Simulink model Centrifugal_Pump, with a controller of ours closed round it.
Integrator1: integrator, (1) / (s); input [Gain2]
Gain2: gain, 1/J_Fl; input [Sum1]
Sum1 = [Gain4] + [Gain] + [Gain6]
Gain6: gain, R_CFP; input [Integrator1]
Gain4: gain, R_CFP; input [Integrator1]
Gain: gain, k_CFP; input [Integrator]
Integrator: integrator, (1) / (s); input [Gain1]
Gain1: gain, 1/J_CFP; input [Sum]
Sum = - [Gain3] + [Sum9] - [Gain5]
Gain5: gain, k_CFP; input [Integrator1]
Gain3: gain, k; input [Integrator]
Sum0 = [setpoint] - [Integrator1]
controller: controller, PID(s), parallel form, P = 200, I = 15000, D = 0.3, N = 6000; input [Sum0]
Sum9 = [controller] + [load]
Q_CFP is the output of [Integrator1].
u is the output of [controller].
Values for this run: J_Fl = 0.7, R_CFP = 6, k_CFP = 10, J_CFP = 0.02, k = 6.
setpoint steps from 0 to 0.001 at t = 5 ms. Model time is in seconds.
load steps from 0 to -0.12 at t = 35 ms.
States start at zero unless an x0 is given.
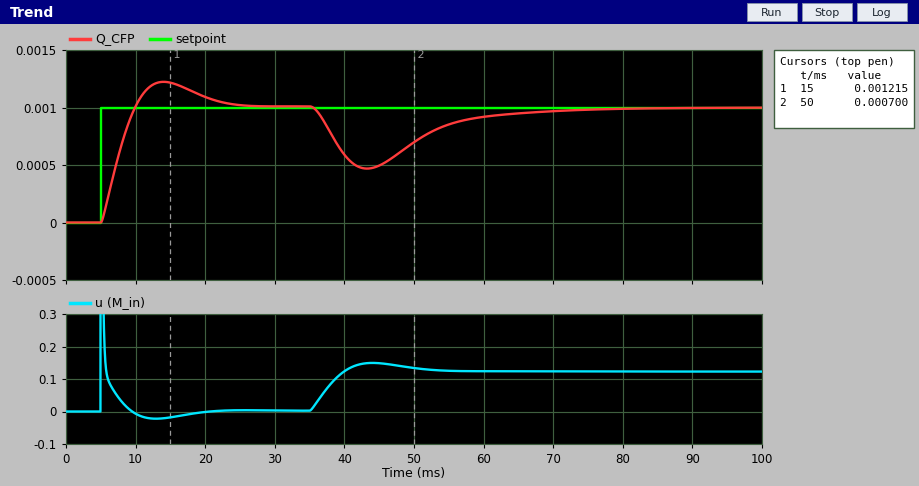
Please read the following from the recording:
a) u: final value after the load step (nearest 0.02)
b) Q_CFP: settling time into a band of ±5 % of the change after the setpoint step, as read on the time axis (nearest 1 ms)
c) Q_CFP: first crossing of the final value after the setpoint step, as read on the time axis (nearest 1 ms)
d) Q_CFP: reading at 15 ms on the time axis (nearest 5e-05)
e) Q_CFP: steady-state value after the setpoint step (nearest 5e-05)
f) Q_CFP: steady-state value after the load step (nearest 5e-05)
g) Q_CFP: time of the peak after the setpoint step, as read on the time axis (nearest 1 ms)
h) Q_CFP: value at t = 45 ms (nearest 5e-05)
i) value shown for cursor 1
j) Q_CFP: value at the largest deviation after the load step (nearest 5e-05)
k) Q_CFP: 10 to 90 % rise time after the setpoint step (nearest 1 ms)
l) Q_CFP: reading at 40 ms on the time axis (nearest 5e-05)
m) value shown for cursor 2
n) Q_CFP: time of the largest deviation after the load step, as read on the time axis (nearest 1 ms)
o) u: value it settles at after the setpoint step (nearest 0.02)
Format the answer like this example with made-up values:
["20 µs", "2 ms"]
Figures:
["0.12", "22 ms", "10 ms", "0.00120", "0.00100", "0.00100", "14 ms", "0.00050", "0.001215", "0.00045", "4 ms", "0.00060", "0.000700", "43 ms", "0.00"]
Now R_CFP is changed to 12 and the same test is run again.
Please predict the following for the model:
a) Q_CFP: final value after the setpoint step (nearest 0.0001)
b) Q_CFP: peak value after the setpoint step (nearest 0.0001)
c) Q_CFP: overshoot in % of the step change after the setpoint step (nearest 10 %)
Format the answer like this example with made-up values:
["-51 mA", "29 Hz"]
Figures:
["0.0010", "0.0013", "30 %"]
